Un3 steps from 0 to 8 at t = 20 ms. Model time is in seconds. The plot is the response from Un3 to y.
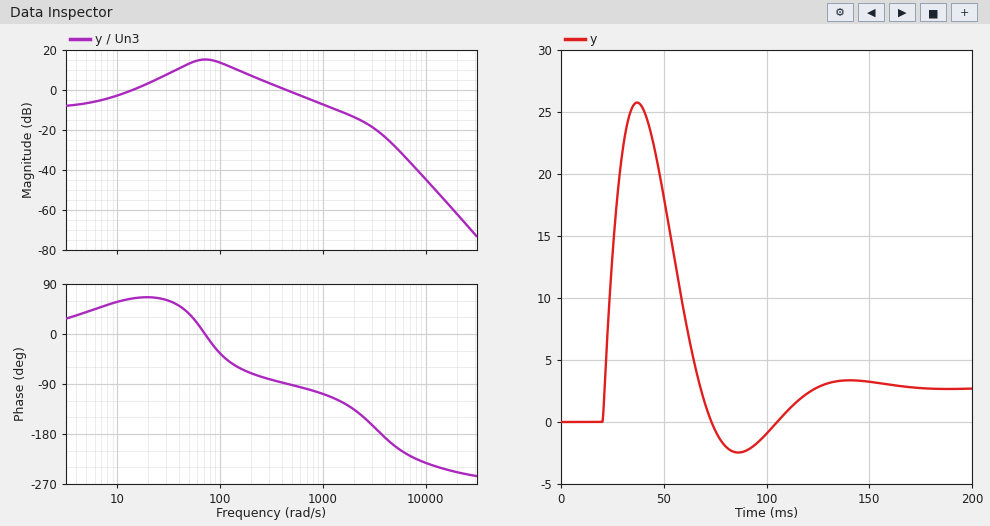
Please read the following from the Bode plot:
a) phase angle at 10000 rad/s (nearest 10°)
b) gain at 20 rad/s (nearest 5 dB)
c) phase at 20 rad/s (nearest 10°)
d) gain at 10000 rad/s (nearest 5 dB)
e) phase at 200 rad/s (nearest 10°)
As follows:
-230°
5 dB
70°
-45 dB
-70°
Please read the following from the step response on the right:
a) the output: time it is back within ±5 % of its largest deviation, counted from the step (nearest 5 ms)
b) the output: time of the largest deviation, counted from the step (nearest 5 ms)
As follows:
95 ms
15 ms
